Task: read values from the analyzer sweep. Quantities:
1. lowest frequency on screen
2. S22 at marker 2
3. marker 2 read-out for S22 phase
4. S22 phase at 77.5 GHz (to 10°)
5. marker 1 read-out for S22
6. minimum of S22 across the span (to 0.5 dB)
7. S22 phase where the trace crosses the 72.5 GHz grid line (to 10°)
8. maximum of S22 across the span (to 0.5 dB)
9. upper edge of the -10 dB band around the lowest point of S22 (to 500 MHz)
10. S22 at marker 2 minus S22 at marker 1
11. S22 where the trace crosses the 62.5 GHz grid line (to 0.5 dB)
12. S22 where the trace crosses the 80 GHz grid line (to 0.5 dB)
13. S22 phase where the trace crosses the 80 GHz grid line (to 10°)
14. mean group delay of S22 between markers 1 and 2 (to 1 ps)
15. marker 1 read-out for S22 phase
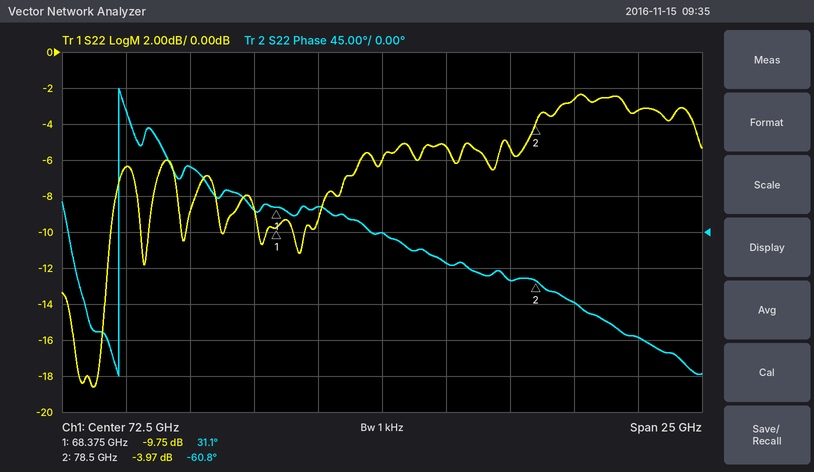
60 GHz
-3.97 dB
-60.8°
-60°
-9.75 dB
-18.5 dB
0°
-2.5 dB
62.0 GHz
5.78 dB
-6.5 dB
-2.5 dB
-90°
25 ps
31.1°
